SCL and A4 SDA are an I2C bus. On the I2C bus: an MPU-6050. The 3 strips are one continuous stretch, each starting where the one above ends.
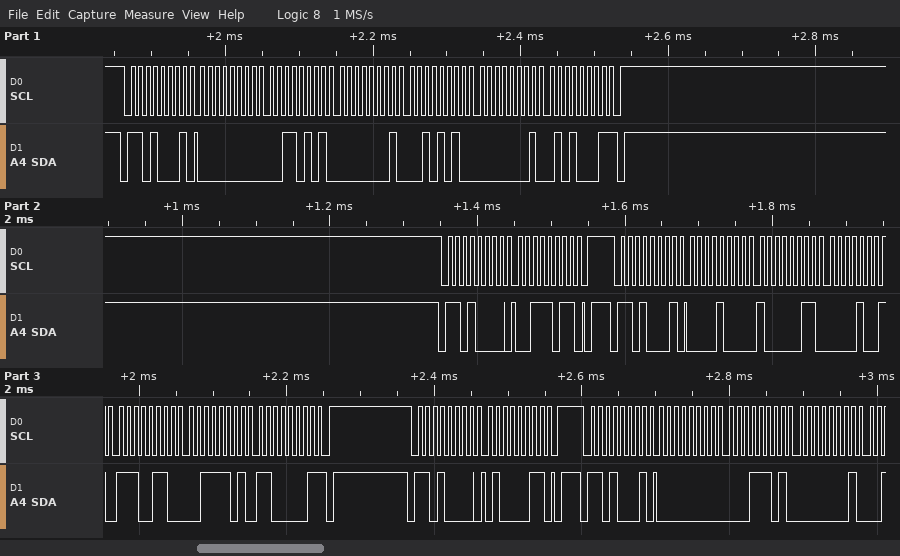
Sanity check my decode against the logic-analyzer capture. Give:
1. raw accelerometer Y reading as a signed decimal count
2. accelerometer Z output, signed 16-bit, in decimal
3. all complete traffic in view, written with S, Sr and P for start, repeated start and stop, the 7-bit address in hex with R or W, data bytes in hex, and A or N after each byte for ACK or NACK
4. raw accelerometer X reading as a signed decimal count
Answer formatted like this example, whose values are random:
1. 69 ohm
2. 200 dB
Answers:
1. 2534
2. 15809
3. S 68R A 00 A 35 A 01 A 2A A 01 A 51 N P S 68W A 3B A P S 68R A 08 A 83 A 09 A E6 A 3D A C1 N P S 68W A 43 A P S 68R A 00 A 1D A 01 A
4. 2179
